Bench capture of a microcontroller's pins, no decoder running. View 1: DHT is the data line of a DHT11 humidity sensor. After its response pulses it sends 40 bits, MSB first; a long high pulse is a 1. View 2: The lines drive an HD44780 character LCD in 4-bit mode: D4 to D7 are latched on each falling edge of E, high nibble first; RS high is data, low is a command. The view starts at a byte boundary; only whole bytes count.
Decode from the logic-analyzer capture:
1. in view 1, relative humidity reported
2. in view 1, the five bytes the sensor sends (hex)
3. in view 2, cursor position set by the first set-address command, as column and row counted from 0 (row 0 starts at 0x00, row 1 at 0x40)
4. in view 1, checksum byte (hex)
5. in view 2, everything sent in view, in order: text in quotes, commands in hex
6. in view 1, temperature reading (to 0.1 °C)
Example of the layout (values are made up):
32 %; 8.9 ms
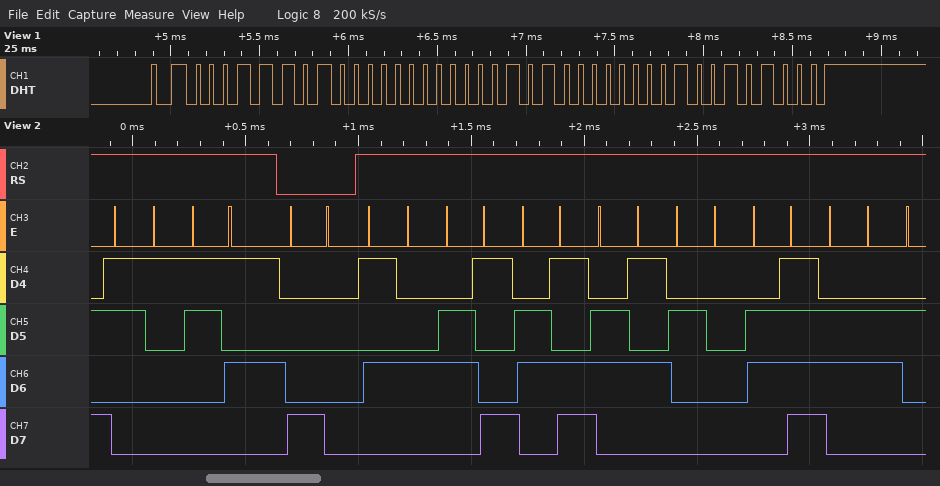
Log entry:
29 %; 1D 00 0A 01 28; column 0, row 0; 0x28; "15" 0x80 "Time of"; 10.1 °C
